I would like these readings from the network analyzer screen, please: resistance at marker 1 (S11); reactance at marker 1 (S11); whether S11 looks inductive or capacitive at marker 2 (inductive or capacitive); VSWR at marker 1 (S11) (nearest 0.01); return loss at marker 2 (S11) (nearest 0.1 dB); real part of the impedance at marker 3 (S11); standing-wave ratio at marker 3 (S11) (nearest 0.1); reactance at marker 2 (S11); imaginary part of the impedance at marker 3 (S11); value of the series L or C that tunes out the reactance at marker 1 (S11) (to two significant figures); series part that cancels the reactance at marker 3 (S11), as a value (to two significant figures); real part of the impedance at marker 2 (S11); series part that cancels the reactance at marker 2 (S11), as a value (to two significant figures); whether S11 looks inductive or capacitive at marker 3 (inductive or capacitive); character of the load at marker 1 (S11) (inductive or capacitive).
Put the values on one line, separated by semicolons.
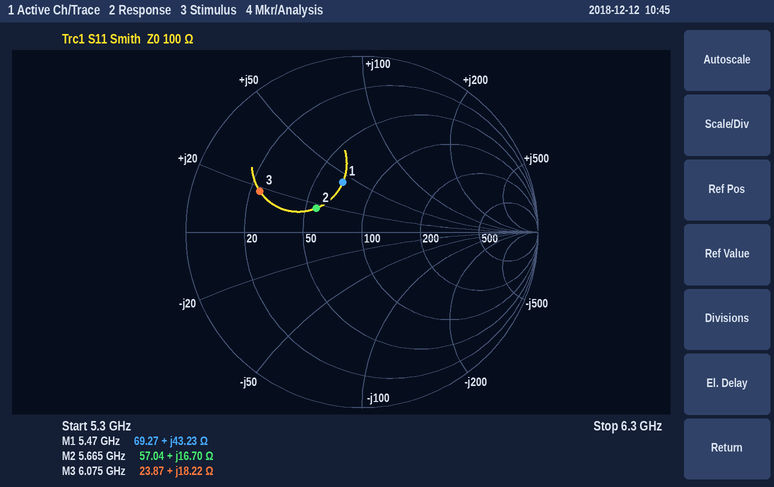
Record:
69.27 Ω; +43.23 Ω; inductive; 1.87; 10.7 dB; 23.87 Ω; 4.3; +16.70 Ω; +18.22 Ω; 670 fF; 1.4 pF; 57.04 Ω; 1.7 pF; inductive; inductive
